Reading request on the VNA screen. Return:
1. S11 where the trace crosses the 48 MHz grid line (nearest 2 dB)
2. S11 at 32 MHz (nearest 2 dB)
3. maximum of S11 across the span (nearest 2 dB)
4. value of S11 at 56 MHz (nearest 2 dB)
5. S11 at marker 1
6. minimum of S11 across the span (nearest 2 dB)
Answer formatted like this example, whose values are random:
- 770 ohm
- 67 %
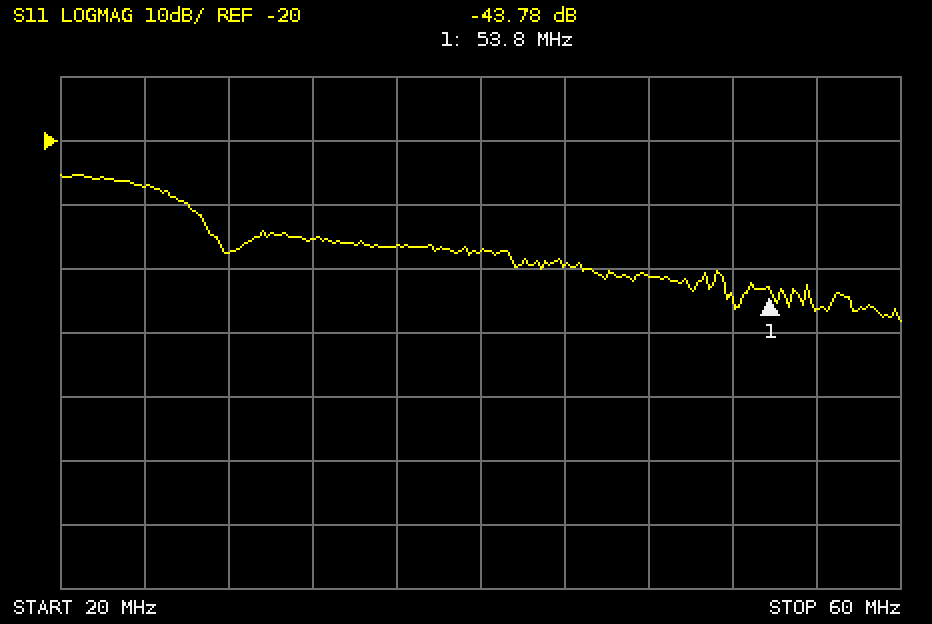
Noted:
- -42 dB
- -36 dB
- -26 dB
- -46 dB
- -43.78 dB
- -48 dB
